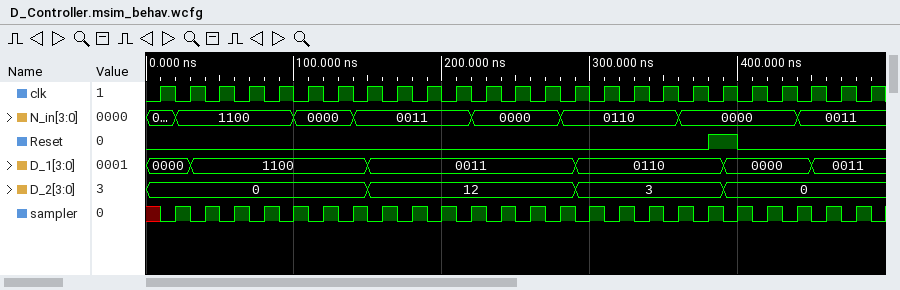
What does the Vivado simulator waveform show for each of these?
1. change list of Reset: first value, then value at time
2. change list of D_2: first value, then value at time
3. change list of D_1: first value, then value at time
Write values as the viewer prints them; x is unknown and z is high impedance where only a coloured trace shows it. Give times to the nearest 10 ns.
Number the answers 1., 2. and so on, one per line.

1. 0, 1 at 380 ns, 0 at 400 ns
2. 0, 12 at 150 ns, 3 at 290 ns, 0 at 390 ns
3. 0000, 1100 at 30 ns, 0011 at 150 ns, 0110 at 290 ns, 0000 at 390 ns, 0011 at 450 ns
